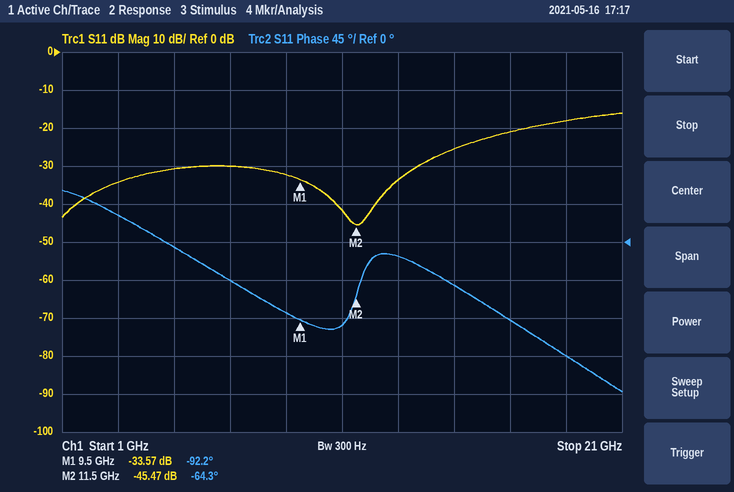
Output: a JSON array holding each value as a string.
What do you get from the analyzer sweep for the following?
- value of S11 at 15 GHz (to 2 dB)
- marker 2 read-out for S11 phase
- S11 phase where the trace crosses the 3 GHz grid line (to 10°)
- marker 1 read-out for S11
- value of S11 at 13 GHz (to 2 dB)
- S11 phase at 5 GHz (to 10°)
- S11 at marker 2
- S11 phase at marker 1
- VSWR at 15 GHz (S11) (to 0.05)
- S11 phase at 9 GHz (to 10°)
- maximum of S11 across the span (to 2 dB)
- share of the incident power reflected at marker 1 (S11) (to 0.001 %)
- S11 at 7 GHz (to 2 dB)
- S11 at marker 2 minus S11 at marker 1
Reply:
["-26 dB", "-64.3°", "30°", "-33.57 dB", "-34 dB", "-10°", "-45.47 dB", "-92.2°", "1.10", "-80°", "-16 dB", "0.044 %", "-30 dB", "-11.90 dB"]
